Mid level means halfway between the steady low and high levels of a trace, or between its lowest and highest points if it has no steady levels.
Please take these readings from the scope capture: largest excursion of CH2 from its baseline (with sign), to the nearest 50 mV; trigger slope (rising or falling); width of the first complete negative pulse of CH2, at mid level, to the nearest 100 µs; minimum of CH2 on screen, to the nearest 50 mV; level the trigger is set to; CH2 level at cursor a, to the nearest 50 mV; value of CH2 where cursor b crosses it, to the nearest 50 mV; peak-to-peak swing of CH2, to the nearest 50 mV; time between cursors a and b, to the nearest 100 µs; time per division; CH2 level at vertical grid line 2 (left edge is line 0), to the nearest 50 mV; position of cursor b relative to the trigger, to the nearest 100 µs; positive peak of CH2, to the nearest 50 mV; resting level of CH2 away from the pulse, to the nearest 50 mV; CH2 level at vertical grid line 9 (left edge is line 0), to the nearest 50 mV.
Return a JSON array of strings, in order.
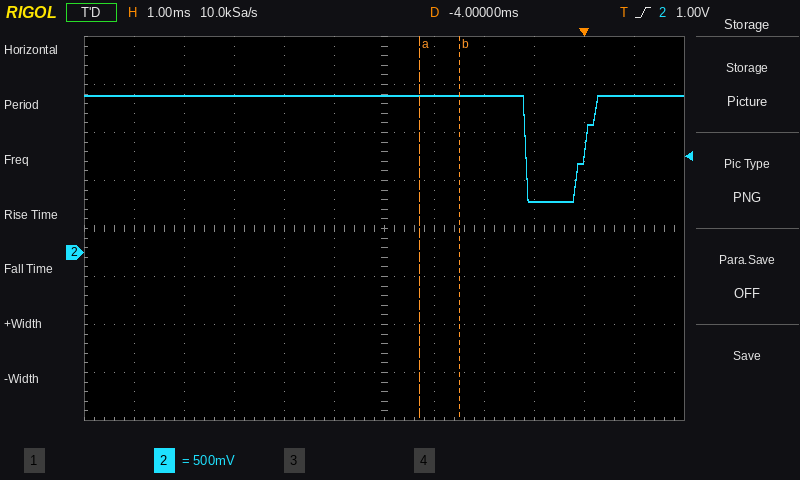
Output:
["-1.10 V", "rising", "1.2 ms", "550 mV", "1.00 V", "1.65 V", "1.65 V", "1.10 V", "800 µs", "1 ms", "1.65 V", "-2.5 ms", "1.65 V", "1.65 V", "550 mV"]
